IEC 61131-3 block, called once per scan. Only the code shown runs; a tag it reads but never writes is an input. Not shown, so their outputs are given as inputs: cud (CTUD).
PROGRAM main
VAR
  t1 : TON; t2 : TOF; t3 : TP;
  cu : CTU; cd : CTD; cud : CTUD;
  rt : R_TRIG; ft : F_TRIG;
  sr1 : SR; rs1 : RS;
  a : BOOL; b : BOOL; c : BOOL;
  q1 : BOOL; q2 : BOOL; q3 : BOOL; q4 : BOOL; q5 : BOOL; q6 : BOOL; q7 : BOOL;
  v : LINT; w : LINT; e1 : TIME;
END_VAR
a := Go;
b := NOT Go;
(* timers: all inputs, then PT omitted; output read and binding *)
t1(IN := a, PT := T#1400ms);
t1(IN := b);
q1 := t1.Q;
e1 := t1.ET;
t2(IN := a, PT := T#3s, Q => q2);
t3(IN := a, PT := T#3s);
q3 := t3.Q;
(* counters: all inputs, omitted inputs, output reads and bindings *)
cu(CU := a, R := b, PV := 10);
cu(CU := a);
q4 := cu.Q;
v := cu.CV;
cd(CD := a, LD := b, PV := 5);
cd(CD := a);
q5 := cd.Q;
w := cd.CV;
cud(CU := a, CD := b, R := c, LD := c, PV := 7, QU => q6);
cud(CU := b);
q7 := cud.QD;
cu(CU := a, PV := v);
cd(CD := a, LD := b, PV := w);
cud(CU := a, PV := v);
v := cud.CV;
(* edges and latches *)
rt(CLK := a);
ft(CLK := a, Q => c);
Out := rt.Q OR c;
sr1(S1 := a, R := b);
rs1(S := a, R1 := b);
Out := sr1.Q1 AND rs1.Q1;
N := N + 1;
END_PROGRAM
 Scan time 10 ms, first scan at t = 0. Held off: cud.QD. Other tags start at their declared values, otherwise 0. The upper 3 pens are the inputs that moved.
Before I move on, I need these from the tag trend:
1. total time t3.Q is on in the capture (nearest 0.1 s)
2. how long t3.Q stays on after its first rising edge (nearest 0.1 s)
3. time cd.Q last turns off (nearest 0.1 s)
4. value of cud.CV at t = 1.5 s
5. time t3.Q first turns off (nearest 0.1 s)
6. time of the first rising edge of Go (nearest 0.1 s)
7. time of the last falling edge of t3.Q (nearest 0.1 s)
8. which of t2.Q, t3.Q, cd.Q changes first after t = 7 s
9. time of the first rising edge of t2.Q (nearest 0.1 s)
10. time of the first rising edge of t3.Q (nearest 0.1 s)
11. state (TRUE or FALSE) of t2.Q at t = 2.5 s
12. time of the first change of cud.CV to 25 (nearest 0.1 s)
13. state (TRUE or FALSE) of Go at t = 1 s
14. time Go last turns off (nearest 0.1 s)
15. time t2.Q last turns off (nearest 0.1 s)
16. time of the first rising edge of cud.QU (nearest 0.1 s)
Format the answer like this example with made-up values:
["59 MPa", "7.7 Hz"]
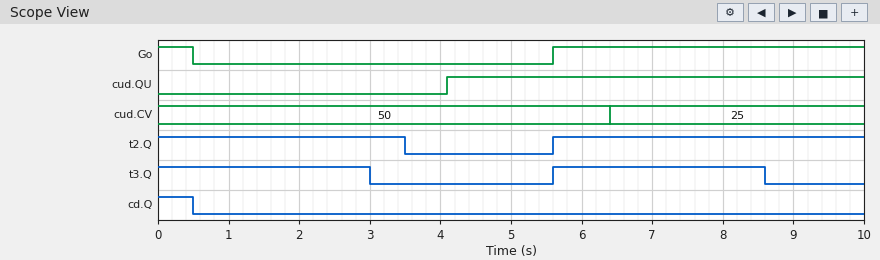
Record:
["6.0 s", "3.0 s", "0.5 s", "50", "3.0 s", "5.6 s", "8.6 s", "t3.Q", "5.6 s", "5.6 s", "TRUE", "6.4 s", "FALSE", "0.5 s", "3.5 s", "4.1 s"]
